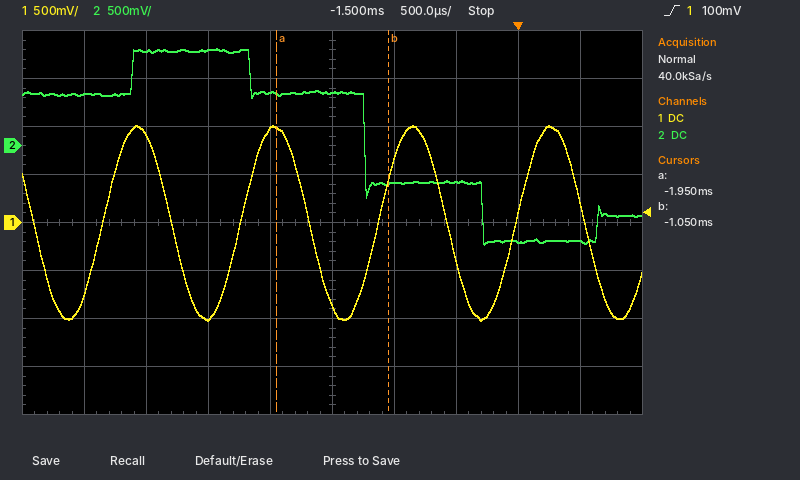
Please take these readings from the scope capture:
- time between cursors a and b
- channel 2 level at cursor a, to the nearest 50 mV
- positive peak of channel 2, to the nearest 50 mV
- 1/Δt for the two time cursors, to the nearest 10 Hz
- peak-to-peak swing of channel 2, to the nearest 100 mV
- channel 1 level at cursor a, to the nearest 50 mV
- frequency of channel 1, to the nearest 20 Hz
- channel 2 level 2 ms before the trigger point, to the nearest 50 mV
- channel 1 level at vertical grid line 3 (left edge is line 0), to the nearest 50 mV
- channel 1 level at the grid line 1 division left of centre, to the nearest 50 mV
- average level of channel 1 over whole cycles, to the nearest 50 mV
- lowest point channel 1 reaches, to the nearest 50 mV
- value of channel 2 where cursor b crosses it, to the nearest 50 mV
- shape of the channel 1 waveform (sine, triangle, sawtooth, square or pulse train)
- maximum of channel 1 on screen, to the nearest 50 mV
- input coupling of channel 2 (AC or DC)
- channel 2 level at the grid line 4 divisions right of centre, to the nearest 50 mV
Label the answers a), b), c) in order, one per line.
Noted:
a) 900 µs
b) 550 mV
c) 1.00 V
d) 1.11 kHz
e) 2.00 V
f) 1.00 V
g) 900 Hz
h) 550 mV
i) -1.00 V
j) 950 mV
k) 0 mV
l) -1.00 V
m) -400 mV
n) sine
o) 1.00 V
p) DC
q) -1.00 V
